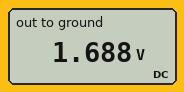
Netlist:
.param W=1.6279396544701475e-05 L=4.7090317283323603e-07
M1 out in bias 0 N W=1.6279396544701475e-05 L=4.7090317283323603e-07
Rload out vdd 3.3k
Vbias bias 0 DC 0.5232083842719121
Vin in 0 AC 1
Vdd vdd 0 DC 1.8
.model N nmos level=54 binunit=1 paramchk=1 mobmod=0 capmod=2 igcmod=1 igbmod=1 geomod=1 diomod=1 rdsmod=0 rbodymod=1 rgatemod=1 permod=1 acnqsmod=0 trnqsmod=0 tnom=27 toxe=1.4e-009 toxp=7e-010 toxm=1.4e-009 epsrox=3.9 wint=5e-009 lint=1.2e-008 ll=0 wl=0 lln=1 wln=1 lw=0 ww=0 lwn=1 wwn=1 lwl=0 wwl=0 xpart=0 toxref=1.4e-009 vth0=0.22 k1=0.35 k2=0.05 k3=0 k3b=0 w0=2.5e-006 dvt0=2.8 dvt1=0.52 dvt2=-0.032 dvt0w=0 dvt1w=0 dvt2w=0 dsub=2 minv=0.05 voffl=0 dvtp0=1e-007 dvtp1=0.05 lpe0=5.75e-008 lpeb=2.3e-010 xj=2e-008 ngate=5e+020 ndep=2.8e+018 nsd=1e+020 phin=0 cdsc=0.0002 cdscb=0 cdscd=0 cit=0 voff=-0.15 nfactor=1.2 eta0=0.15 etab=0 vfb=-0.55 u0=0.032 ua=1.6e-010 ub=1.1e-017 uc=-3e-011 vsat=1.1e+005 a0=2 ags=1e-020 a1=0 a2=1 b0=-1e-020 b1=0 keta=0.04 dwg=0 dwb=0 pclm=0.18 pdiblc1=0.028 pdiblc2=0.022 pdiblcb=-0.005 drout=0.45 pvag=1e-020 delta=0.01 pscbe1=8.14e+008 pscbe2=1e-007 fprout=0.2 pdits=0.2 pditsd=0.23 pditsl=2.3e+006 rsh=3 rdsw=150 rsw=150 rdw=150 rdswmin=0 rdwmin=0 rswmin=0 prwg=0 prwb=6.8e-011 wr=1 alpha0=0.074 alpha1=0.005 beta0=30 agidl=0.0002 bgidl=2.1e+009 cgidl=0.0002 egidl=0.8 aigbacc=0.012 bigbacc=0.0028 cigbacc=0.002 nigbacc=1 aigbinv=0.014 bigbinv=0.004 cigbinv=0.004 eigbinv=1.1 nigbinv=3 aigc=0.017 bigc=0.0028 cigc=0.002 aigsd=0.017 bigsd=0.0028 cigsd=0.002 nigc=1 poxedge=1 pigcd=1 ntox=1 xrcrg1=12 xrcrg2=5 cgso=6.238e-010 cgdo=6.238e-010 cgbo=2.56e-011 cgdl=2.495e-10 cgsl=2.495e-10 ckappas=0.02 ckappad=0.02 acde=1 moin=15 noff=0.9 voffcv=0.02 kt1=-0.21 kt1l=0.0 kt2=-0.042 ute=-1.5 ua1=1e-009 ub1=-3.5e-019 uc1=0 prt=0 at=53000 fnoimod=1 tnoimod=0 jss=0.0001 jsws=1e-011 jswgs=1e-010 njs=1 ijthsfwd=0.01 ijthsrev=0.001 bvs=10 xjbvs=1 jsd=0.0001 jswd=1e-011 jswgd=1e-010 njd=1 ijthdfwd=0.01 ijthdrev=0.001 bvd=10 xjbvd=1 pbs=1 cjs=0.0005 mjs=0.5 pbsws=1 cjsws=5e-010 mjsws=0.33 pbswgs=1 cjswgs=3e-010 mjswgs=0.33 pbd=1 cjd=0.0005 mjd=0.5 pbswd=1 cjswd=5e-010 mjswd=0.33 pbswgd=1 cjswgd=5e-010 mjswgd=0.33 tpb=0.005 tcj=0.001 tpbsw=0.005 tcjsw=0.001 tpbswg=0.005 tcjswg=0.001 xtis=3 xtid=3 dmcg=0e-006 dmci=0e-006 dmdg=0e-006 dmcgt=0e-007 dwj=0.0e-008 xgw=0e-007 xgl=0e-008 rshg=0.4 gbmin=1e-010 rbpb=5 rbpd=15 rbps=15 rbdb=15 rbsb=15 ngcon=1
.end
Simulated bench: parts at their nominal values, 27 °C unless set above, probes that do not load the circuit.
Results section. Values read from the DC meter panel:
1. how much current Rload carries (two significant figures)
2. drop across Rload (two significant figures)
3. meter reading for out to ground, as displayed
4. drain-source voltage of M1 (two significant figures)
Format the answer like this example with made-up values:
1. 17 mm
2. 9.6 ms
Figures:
1. 34 µA
2. 110 mV
3. 1.688 V
4. 1.2 V
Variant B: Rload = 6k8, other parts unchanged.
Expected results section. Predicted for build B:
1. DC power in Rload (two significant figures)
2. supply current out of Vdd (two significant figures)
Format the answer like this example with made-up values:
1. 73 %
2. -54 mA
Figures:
1. 3.2 µW
2. 22 µA
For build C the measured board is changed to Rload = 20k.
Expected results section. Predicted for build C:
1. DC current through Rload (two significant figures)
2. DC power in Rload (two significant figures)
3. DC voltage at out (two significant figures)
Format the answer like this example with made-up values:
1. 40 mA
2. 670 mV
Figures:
1. 10 µA
2. 2.0 µW
3. 1.6 V
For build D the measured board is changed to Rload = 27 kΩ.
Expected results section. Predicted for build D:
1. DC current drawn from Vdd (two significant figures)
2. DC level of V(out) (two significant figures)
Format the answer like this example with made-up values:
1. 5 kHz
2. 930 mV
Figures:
1. 8.0 µA
2. 1.6 V
